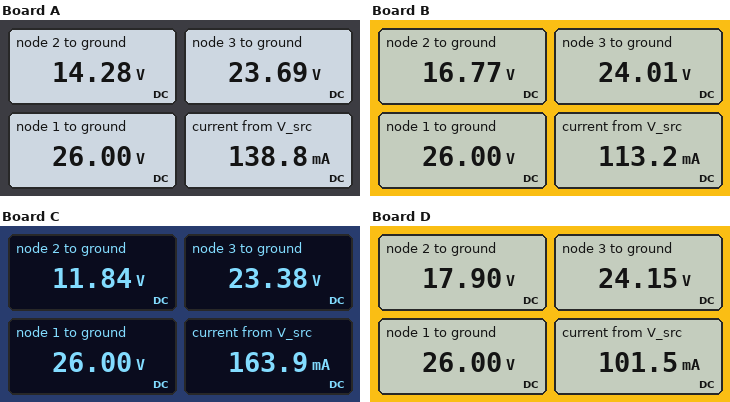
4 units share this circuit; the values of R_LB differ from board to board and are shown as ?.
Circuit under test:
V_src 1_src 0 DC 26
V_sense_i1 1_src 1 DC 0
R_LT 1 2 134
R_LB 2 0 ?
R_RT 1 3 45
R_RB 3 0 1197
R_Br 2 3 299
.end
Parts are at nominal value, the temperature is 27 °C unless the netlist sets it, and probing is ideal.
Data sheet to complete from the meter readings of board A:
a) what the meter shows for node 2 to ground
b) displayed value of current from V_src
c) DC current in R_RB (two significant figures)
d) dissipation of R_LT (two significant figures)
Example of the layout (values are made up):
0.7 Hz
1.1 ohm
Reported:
14.28 V
138.8 mA
20 mA
1.0 W
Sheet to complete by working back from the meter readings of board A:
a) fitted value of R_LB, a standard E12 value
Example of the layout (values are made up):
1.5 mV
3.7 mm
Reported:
120 Ω
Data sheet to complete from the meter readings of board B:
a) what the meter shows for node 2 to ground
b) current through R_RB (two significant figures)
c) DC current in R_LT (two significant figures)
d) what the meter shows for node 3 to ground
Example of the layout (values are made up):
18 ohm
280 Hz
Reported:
16.77 V
20 mA
69 mA
24.01 V
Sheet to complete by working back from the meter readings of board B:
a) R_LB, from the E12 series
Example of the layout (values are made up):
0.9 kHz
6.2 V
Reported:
180 Ω
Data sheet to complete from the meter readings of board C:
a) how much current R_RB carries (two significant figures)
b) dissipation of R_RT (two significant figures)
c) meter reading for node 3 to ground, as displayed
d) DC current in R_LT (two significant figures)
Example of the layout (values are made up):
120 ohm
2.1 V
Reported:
20 mA
150 mW
23.38 V
110 mA
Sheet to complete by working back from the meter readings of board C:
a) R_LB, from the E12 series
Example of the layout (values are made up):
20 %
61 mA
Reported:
82 Ω
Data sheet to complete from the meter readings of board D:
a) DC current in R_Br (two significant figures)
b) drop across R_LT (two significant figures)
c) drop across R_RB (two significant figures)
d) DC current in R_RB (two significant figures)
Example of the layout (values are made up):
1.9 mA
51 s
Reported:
21 mA
8.1 V
24 V
20 mA
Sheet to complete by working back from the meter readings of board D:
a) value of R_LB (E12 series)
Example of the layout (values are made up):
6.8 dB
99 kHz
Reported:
220 Ω
